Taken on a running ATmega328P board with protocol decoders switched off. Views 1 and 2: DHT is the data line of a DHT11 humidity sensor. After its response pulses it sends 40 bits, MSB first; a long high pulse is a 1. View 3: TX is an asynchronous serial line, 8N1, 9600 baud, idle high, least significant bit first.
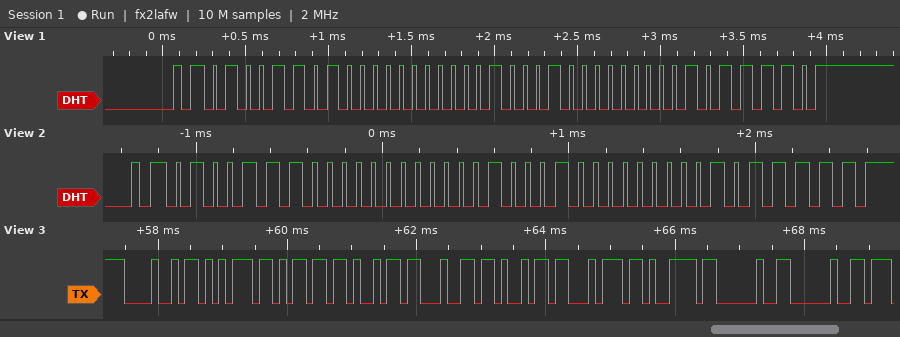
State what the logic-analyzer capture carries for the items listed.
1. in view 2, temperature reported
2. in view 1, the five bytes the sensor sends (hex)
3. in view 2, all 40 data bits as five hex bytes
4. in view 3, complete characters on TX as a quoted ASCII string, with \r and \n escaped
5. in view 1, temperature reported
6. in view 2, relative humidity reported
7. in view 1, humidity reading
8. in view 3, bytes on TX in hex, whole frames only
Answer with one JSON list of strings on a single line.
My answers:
["17.0 °C", "4D 00 11 00 5E", "4E 00 11 00 5F", "\"Humidity  \"", "17.0 °C", "78 %", "77 %", "0x48 0x75 0x6D 0x69 0x64 0x69 0x74 0x79 0x20 0x20"]
